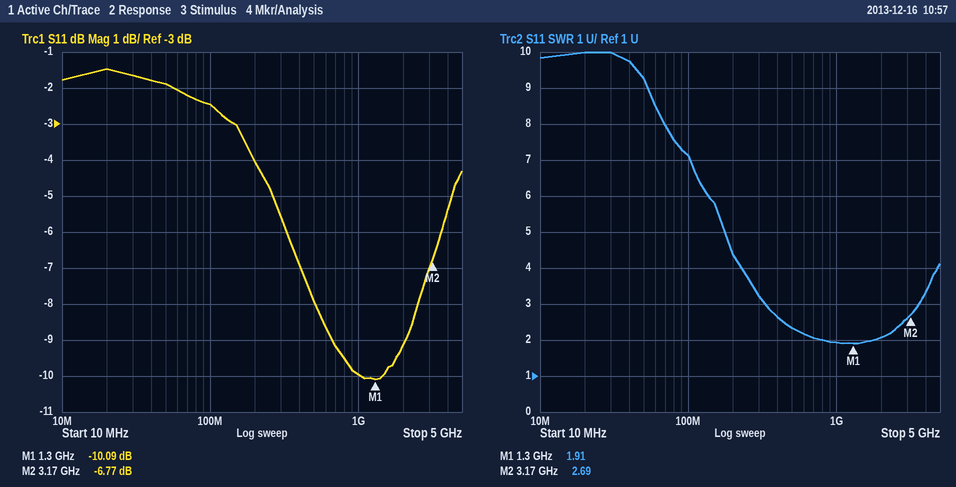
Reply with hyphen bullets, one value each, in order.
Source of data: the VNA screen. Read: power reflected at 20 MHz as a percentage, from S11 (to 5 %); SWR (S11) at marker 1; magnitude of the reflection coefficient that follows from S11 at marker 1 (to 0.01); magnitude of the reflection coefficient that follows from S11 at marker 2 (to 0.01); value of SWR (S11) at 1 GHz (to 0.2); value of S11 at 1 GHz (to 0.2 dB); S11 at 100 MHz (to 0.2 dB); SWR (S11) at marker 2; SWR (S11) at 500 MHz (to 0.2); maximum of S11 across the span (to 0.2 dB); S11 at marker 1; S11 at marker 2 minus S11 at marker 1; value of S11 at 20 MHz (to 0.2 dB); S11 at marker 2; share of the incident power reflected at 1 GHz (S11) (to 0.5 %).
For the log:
- 70 %
- 1.91
- 0.31
- 0.46
- 2.0
- -10.0 dB
- -2.4 dB
- 2.69
- 2.4
- -1.4 dB
- -10.09 dB
- 3.32 dB
- -1.4 dB
- -6.77 dB
- 10.0 %
